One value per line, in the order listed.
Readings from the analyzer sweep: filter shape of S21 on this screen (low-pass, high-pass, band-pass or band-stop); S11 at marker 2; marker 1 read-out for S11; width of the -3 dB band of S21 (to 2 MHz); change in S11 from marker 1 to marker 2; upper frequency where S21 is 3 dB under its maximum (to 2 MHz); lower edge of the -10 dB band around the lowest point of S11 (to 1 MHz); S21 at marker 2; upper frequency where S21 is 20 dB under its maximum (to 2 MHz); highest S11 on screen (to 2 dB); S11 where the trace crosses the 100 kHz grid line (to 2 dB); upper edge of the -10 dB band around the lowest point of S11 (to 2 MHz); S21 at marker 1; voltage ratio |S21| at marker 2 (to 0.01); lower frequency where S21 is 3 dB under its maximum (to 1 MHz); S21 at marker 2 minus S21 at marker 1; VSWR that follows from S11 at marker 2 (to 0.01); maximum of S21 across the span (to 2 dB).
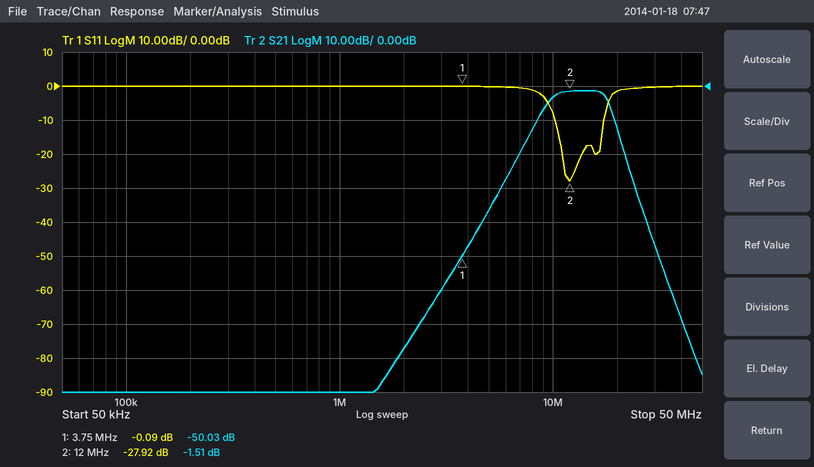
band-pass
-27.92 dB
-0.09 dB
8 MHz
-27.83 dB
18 MHz
10 MHz
-1.51 dB
22 MHz
0 dB
0 dB
18 MHz
-50.03 dB
0.84
10 MHz
48.52 dB
1.08
-2 dB
